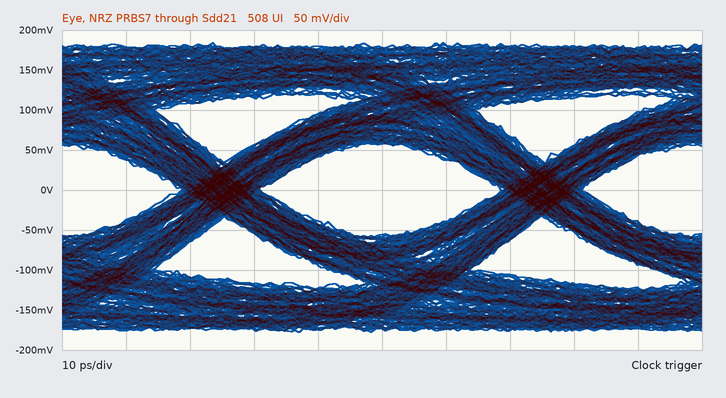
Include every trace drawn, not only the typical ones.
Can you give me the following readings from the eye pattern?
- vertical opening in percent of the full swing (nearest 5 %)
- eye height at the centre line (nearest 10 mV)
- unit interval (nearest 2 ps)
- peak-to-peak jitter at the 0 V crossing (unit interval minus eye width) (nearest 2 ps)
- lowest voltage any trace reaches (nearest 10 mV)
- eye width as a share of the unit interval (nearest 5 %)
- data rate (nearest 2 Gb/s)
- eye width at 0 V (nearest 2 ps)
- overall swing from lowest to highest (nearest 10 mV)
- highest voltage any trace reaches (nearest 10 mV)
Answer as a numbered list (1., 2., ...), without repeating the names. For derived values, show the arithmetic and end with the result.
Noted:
1. 110 mV / 360 mV ≈ 30.6 %, so 30 % to the nearest 5 %
2. 110 mV
3. 50 ps
4. 12 ps
5. -180 mV
6. 38 ps / 50 ps ≈ 76.0 %, so 75 % to the nearest 5 %
7. 20 Gb/s
8. 38 ps
9. 360 mV
10. 180 mV
